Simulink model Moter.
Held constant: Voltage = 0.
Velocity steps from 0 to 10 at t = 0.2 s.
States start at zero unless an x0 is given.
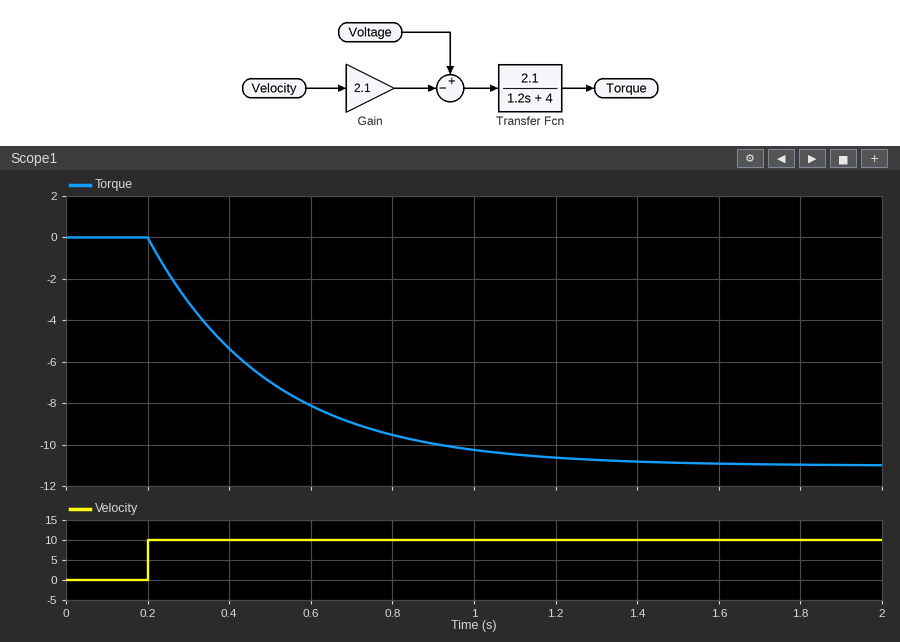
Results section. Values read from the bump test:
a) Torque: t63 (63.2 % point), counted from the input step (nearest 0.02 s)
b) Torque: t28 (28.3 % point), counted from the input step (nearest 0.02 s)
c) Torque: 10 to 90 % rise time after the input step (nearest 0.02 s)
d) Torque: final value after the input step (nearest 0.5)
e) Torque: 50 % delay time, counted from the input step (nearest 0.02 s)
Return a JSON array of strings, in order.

["0.30 s", "0.10 s", "0.66 s", "-11.0", "0.20 s"]
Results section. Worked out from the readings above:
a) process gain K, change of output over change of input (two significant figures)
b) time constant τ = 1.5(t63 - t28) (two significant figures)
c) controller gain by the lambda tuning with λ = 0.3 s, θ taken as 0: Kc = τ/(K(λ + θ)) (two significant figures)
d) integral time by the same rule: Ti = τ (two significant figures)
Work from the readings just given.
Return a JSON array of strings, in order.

["-1.1", "0.30 s", "-0.91", "0.30 s"]
